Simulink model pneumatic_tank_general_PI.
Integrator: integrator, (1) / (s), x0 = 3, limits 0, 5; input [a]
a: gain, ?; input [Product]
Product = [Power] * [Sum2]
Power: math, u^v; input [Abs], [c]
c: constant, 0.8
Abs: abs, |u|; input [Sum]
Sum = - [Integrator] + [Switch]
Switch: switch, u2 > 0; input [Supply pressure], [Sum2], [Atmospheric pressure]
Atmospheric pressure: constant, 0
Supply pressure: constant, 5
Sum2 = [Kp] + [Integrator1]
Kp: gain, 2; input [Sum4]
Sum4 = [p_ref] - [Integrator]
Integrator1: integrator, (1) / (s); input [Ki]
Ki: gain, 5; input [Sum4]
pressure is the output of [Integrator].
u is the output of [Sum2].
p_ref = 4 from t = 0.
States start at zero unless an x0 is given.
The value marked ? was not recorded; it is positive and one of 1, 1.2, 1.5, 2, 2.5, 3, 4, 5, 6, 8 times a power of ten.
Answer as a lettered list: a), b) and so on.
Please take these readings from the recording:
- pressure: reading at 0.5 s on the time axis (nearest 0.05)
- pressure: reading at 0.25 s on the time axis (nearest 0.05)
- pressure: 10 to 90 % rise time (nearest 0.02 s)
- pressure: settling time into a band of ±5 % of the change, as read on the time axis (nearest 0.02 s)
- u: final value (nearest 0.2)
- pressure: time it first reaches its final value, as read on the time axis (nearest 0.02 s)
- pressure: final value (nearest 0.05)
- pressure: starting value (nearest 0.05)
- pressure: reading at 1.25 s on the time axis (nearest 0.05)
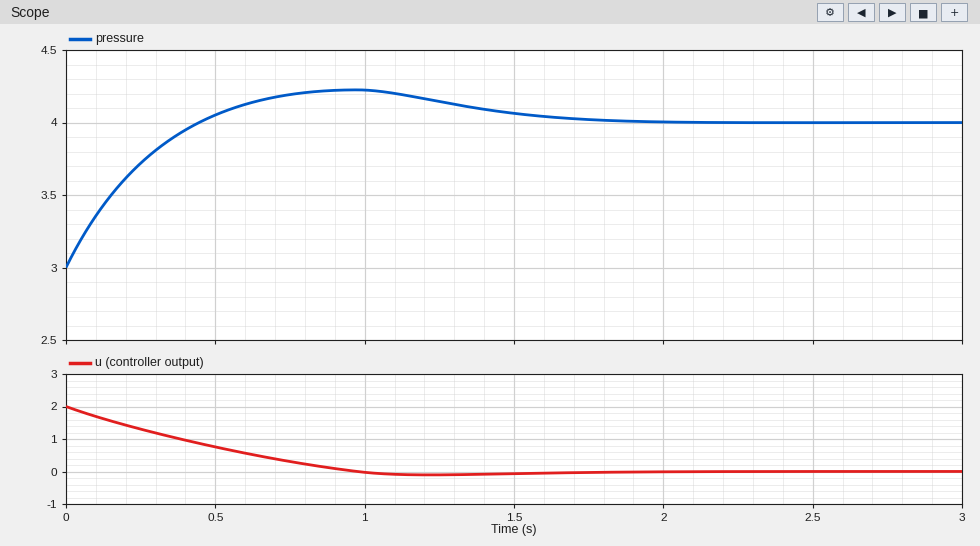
a) 4.05
b) 3.70
c) 0.34 s
d) 1.56 s
e) 0.0
f) 0.44 s
g) 4.00
h) 3.00
i) 4.15
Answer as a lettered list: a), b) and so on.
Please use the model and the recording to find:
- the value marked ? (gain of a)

a) 1.2
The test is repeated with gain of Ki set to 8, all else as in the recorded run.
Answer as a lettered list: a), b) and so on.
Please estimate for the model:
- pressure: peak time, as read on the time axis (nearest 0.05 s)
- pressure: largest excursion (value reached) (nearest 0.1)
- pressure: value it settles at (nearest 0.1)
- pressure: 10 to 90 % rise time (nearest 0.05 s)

a) 0.80 s
b) 4.3
c) 4.0
d) 0.30 s
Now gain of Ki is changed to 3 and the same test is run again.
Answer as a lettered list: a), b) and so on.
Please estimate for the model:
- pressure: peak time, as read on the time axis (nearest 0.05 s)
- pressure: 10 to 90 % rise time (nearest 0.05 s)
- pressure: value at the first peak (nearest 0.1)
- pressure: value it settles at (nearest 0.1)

a) 1.20 s
b) 0.40 s
c) 4.2
d) 4.0
